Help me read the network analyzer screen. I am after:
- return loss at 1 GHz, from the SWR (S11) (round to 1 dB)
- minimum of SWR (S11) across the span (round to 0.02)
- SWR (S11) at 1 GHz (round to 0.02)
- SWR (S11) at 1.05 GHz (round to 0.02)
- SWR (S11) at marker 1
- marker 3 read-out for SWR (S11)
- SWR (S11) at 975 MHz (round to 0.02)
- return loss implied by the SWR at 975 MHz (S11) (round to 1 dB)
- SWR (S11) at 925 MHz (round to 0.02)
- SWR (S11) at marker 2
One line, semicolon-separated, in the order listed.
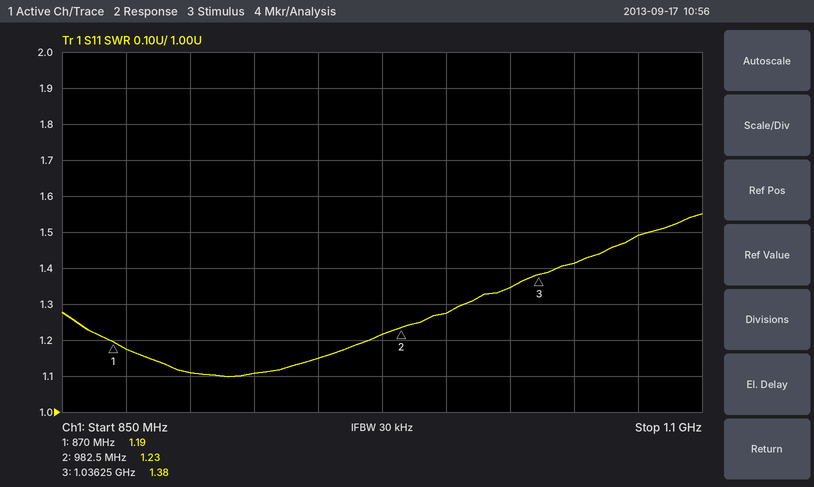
18 dB; 1.10; 1.28; 1.42; 1.19; 1.38; 1.22; 20 dB; 1.10; 1.23
